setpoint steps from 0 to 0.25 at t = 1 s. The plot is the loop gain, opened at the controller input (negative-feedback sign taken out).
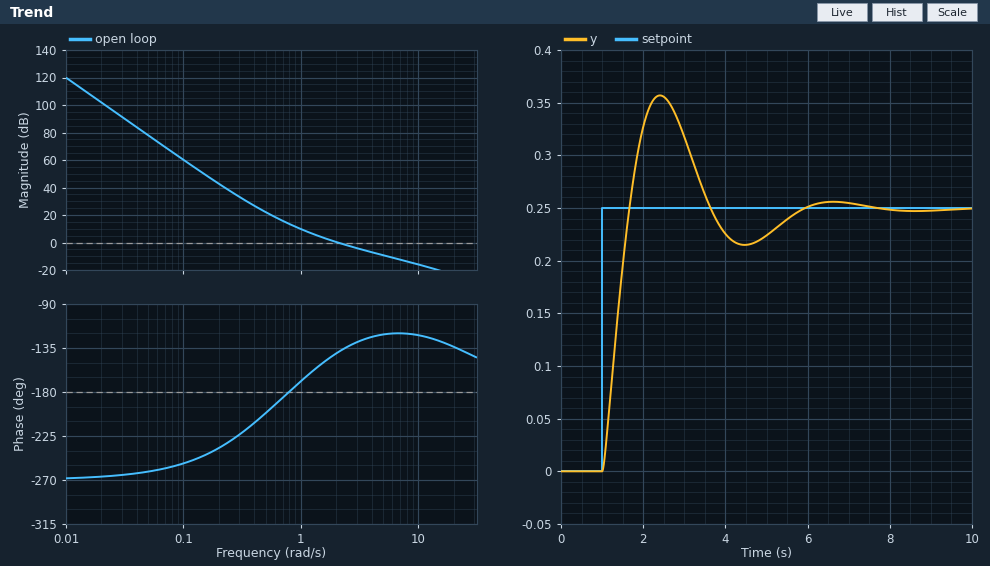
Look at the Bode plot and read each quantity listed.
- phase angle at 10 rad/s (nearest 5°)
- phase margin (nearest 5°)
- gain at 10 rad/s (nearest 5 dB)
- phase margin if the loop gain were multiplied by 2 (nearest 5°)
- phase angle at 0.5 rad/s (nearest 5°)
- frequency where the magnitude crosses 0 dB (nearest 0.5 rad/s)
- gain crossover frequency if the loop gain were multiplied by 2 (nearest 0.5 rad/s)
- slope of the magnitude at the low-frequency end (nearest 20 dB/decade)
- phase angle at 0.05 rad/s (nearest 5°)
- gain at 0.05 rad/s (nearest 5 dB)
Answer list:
-120°
40°
-15 dB
55°
-200°
2.0 rad/s
3.5 rad/s
-60 dB/decade
-260°
80 dB
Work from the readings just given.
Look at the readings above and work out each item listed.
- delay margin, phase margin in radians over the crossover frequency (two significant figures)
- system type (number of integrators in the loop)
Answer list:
0.35 s
3
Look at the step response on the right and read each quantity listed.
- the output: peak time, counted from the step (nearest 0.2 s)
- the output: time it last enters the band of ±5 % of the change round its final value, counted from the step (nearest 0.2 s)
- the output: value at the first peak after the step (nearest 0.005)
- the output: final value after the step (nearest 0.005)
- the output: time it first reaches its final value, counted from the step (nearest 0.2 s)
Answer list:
1.4 s
4.4 s
0.355
0.250
0.6 s
